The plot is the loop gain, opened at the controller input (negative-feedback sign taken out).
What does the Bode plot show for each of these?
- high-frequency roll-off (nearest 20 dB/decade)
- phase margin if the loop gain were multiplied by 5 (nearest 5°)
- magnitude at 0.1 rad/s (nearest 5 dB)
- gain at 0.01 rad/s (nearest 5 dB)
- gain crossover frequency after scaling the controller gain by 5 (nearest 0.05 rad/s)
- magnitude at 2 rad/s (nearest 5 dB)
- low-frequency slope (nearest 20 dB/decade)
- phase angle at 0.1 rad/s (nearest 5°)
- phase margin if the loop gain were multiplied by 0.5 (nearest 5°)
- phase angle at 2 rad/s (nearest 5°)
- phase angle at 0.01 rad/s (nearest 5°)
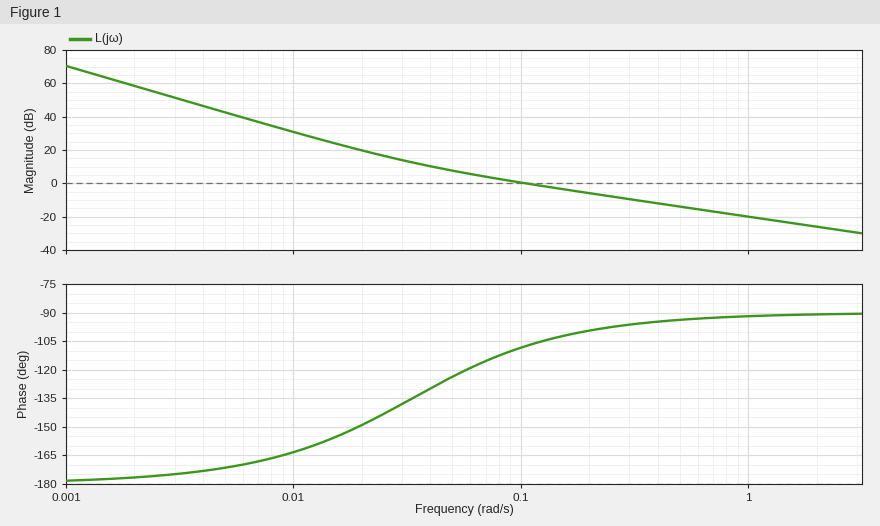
-20 dB/decade
85°
0 dB
30 dB
0.50 rad/s
-25 dB
-40 dB/decade
-110°
60°
-90°
-165°
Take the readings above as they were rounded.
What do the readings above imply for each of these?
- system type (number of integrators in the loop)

2
